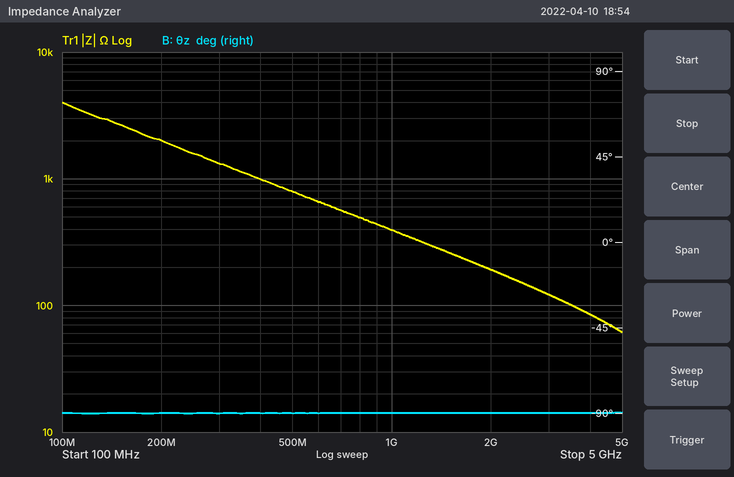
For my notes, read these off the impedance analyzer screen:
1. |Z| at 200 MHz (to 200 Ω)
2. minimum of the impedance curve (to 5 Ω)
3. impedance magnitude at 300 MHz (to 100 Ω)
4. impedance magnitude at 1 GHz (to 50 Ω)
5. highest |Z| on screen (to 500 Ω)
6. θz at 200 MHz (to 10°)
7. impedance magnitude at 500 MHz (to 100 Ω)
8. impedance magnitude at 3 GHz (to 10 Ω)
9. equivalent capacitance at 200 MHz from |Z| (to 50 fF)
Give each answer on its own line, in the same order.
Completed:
2.0 kΩ
60 Ω
1.3 kΩ
400 Ω
4.0 kΩ
-90°
800 Ω
120 Ω
400 fF
